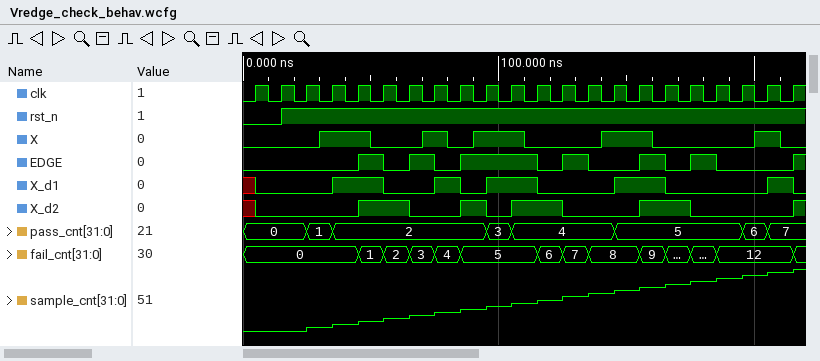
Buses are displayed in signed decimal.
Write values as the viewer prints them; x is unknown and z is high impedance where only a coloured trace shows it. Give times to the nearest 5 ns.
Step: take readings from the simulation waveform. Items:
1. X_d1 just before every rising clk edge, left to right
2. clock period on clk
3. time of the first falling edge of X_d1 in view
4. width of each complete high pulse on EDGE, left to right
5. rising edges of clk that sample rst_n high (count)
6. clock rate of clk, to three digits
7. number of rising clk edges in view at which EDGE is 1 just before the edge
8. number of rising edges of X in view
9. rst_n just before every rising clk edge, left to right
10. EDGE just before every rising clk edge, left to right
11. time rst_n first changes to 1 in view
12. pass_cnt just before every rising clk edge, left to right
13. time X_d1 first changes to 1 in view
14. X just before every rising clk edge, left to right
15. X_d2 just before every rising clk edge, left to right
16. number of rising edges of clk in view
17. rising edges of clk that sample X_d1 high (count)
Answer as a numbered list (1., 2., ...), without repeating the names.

1. x 0 0 0 1 1 0 0 1 0 1 1 0 0 0 1 1 0 0 0 0 1
2. 10 ns
3. 55 ns
4. 10 ns, 10 ns, 30 ns, 10 ns, 10 ns, 10 ns
5. 20
6. 100 MHz
7. 8
8. 5
9. 0 0 1 1 1 1 1 1 1 1 1 1 1 1 1 1 1 1 1 1 1 1
10. 0 0 0 0 0 1 0 1 0 1 1 1 0 1 0 0 1 0 1 0 0 0
11. 15 ns
12. 0, 0, 0, 1, 2, 2, 2, 2, 2, 2, 3, 4, 4, 4, 4, 5, 5, 5, 5, 5, 6, 7
13. 35 ns
14. 0 0 0 1 1 0 0 1 0 1 1 0 0 0 1 1 0 0 0 0 1 0
15. x 0 0 0 0 1 1 0 0 1 0 1 1 0 0 0 1 1 0 0 0 0
16. 22
17. 8
